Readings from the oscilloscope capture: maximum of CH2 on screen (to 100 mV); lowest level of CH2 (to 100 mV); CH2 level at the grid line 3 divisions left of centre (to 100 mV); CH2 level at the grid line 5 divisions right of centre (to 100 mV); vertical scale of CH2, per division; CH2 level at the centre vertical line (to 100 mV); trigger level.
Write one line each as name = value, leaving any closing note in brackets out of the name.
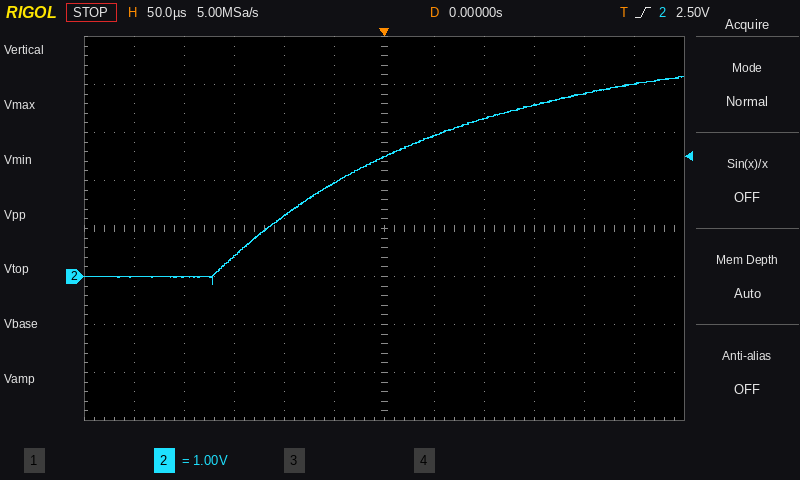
maximum of CH2 on screen = 4.2 V
lowest level of CH2 = -200 mV
CH2 level at the grid line 3 divisions left of centre = 400 mV
CH2 level at the grid line 5 divisions right of centre = 4.0 V
vertical scale of CH2, per division = 1 V
CH2 level at the centre vertical line = 2.5 V
trigger level = 2.50 V
